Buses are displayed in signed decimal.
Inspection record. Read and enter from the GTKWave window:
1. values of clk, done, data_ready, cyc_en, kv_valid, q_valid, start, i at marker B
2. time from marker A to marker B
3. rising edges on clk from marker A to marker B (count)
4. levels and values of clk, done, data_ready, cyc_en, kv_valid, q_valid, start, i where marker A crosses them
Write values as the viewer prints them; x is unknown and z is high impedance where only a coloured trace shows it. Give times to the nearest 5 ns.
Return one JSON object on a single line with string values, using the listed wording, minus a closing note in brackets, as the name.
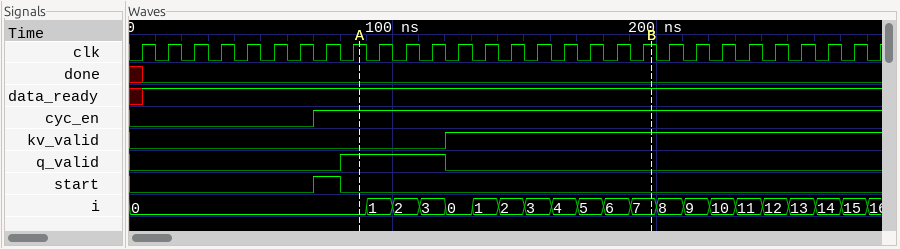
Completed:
{"values of clk, done, data_ready, cyc_en, kv_valid, q_valid, start, i at marker B": "clk=1, done=0, data_ready=1, cyc_en=1, kv_valid=1, q_valid=0, start=0, i=7", "time from marker A to marker B": "110 ns", "rising edges on clk from marker A to marker B": "11", "levels and values of clk, done, data_ready, cyc_en, kv_valid, q_valid, start, i where marker A crosses them": "clk=1, done=0, data_ready=1, cyc_en=1, kv_valid=0, q_valid=1, start=0, i=0"}
